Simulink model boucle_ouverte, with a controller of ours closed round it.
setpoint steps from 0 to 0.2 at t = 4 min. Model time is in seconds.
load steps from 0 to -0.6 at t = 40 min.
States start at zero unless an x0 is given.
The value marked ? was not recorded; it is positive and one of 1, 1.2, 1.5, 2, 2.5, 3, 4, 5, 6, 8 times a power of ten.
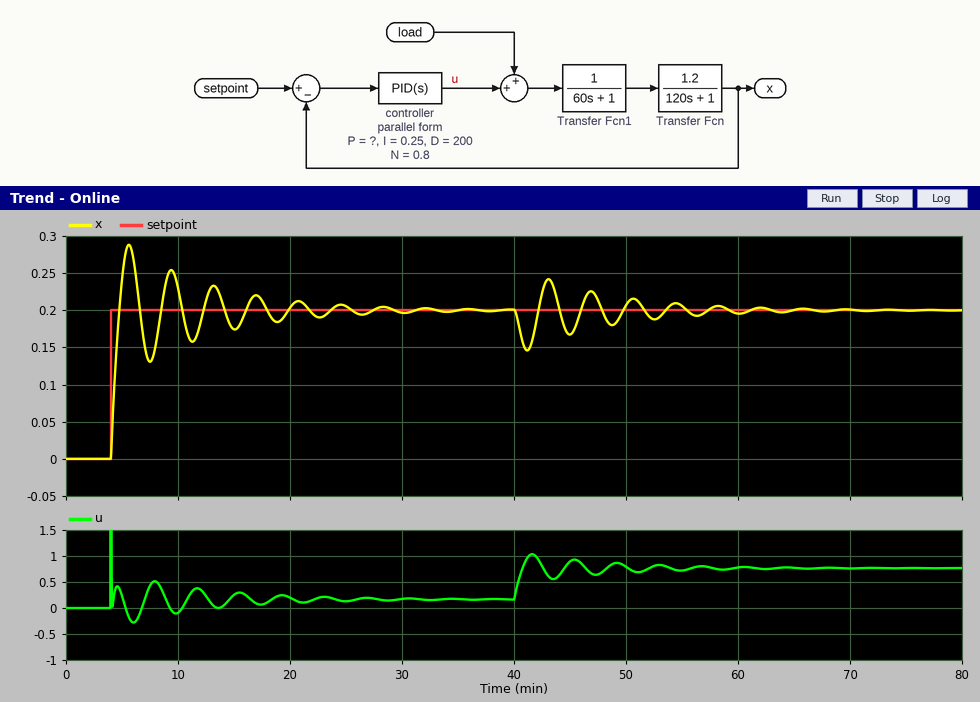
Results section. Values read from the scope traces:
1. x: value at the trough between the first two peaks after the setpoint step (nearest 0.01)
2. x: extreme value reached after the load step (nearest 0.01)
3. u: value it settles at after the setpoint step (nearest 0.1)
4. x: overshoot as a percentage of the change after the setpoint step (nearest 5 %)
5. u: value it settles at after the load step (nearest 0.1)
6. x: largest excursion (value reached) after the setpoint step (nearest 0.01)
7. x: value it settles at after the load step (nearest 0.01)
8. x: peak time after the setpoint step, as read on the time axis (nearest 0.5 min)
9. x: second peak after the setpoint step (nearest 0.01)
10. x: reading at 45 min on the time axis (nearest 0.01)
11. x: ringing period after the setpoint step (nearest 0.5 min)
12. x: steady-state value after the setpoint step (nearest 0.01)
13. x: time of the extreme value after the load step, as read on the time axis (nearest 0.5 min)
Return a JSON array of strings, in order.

["0.13", "0.15", "0.2", "45 %", "0.8", "0.29", "0.20", "5.5 min", "0.25", "0.17", "4.0 min", "0.20", "41.0 min"]
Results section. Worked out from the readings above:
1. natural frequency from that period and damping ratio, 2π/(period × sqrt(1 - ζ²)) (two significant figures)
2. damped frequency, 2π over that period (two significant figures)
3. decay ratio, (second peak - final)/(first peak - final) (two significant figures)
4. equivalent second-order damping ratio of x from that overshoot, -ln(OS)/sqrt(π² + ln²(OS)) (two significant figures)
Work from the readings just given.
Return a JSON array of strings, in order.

["1.6 rad/min", "1.6 rad/min", "0.56", "0.25"]
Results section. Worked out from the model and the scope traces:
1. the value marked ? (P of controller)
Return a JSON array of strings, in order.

["5"]
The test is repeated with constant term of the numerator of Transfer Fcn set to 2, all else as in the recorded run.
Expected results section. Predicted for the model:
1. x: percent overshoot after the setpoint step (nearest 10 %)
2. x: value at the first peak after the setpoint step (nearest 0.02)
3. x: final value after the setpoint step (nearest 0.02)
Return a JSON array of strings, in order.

["30 %", "0.26", "0.20"]
